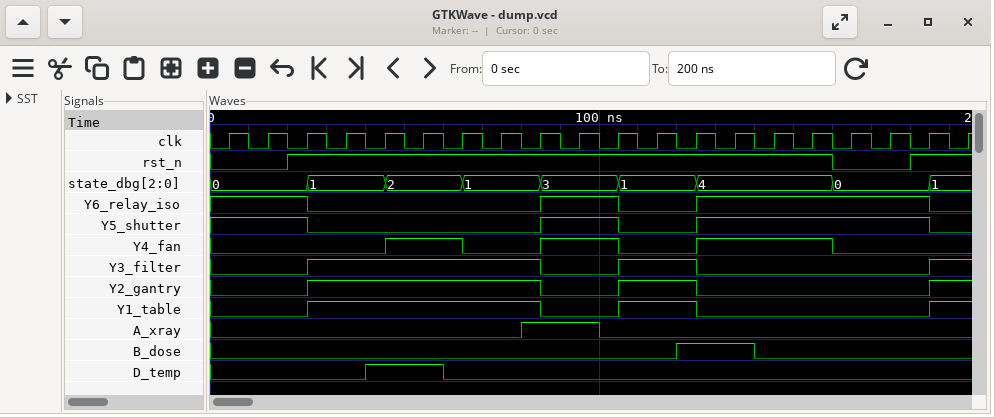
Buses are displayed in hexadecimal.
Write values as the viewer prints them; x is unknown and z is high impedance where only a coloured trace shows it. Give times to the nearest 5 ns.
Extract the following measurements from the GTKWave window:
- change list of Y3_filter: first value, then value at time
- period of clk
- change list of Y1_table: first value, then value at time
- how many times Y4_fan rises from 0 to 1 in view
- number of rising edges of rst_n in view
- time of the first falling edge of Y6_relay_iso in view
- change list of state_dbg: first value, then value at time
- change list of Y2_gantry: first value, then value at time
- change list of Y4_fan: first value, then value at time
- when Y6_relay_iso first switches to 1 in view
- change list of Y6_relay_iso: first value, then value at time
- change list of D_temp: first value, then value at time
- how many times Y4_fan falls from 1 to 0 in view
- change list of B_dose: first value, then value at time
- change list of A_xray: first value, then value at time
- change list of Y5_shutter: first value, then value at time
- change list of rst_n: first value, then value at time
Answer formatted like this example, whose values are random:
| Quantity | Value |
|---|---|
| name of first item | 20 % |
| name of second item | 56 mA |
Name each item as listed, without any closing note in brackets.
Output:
| Quantity | Value |
|---|---|
| change list of Y3_filter: first value, then value at time | 0, 1 at 25 ns, 0 at 85 ns, 1 at 105 ns, 0 at 125 ns, 1 at 185 ns |
| period of clk | 10 ns |
| change list of Y1_table: first value, then value at time | 0, 1 at 25 ns, 0 at 85 ns, 1 at 105 ns, 0 at 125 ns, 1 at 185 ns |
| how many times Y4_fan rises from 0 to 1 in view | 3 |
| number of rising edges of rst_n in view | 2 |
| time of the first falling edge of Y6_relay_iso in view | 25 ns |
| change list of state_dbg: first value, then value at time | 0, 1 at 25 ns, 2 at 45 ns, 1 at 65 ns, 3 at 85 ns, 1 at 105 ns, 4 at 125 ns, 0 at 160 ns, 1 at 185 ns |
| change list of Y2_gantry: first value, then value at time | 0, 1 at 25 ns, 0 at 85 ns, 1 at 105 ns, 0 at 125 ns, 1 at 185 ns |
| change list of Y4_fan: first value, then value at time | 0, 1 at 45 ns, 0 at 65 ns, 1 at 85 ns, 0 at 105 ns, 1 at 125 ns, 0 at 160 ns |
| when Y6_relay_iso first switches to 1 in view | 85 ns |
| change list of Y6_relay_iso: first value, then value at time | 1, 0 at 25 ns, 1 at 85 ns, 0 at 105 ns, 1 at 125 ns, 0 at 185 ns |
| change list of D_temp: first value, then value at time | 0, 1 at 40 ns, 0 at 60 ns |
| how many times Y4_fan falls from 1 to 0 in view | 3 |
| change list of B_dose: first value, then value at time | 0, 1 at 120 ns, 0 at 140 ns |
| change list of A_xray: first value, then value at time | 0, 1 at 80 ns, 0 at 100 ns |
| change list of Y5_shutter: first value, then value at time | 1, 0 at 25 ns, 1 at 85 ns, 0 at 105 ns, 1 at 125 ns, 0 at 185 ns |
| change list of rst_n: first value, then value at time | 0, 1 at 20 ns, 0 at 160 ns, 1 at 180 ns |
